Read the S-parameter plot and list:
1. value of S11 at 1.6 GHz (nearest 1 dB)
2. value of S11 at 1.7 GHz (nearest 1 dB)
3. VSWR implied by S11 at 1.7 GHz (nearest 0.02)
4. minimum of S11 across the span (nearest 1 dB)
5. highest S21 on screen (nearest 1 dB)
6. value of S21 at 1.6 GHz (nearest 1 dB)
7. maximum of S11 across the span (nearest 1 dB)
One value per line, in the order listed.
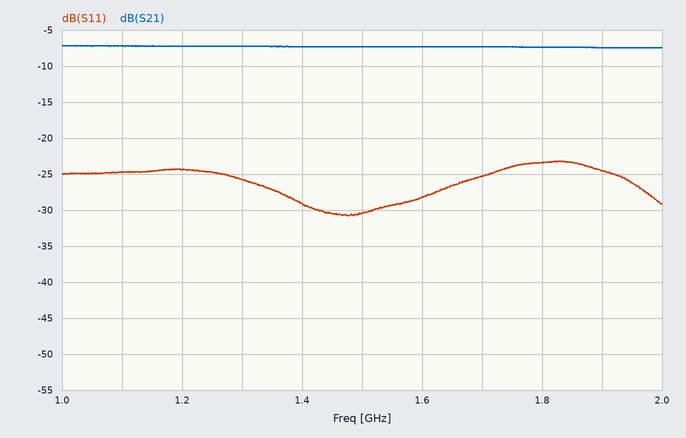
-28 dB
-25 dB
1.12
-31 dB
-7 dB
-7 dB
-23 dB
